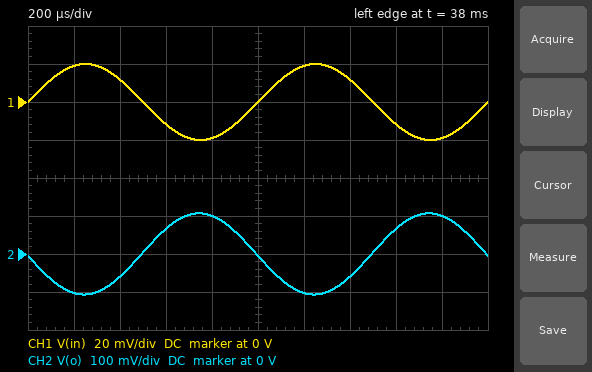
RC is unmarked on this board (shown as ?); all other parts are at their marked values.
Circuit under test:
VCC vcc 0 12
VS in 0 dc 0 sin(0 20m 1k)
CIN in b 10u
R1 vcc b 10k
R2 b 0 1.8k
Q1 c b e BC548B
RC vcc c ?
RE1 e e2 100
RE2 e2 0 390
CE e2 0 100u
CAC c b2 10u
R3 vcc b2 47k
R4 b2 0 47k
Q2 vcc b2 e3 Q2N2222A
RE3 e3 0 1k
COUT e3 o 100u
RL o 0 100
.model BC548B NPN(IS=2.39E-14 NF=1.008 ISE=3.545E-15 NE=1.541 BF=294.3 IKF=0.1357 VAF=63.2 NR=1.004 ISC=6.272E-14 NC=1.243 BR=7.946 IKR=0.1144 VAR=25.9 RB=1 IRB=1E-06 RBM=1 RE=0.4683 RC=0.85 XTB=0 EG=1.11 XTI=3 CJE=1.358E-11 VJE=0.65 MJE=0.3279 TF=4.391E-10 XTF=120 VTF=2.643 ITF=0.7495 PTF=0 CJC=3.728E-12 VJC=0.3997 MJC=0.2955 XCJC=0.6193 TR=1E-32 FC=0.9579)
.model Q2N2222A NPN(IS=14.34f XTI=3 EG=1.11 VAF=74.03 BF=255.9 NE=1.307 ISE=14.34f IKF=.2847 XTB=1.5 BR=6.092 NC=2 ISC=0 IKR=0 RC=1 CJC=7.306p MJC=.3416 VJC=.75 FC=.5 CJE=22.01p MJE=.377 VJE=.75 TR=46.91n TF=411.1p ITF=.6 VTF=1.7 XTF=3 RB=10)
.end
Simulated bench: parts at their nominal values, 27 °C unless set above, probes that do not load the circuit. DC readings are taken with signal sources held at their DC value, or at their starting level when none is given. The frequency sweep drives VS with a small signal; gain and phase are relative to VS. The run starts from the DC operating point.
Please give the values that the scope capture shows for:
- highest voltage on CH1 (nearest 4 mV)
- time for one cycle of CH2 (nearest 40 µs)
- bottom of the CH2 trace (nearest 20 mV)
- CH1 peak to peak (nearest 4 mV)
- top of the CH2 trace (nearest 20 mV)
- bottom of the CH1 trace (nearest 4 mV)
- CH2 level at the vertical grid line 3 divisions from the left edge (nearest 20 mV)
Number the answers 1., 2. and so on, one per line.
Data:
1. 20 mV
2. 1.00 ms
3. -100 mV
4. 40 mV
5. 100 mV
6. -20 mV
7. 60 mV
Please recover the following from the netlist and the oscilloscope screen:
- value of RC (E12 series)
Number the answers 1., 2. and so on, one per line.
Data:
1. 680 Ω
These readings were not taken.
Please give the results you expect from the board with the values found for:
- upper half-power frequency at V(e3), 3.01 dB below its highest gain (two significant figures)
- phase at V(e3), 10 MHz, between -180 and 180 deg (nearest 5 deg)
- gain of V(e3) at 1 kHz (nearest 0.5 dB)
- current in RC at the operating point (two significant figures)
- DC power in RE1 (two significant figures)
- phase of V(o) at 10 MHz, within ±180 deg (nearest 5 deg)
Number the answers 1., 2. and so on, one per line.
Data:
1. 21 MHz
2. 150 deg
3. 14.5 dB
4. 2.4 mA
5. 560 µW
6. 150 deg
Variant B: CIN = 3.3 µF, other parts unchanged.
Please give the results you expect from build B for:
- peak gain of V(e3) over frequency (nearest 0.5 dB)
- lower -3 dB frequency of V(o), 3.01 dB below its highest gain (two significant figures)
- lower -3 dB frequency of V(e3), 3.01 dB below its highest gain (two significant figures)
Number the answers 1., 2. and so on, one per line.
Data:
1. 14.5 dB
2. 45 Hz
3. 40 Hz
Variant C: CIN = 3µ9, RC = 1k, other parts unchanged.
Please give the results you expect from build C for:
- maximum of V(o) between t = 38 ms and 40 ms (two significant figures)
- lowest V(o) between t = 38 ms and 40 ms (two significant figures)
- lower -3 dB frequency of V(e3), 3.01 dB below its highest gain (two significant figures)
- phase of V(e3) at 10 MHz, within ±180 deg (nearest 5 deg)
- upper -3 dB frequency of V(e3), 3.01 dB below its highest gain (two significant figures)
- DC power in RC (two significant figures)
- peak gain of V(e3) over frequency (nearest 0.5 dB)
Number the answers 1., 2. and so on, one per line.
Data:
1. 150 mV
2. -150 mV
3. 36 Hz
4. 145 deg
5. 15 MHz
6. 5.6 mW
7. 17.5 dB
